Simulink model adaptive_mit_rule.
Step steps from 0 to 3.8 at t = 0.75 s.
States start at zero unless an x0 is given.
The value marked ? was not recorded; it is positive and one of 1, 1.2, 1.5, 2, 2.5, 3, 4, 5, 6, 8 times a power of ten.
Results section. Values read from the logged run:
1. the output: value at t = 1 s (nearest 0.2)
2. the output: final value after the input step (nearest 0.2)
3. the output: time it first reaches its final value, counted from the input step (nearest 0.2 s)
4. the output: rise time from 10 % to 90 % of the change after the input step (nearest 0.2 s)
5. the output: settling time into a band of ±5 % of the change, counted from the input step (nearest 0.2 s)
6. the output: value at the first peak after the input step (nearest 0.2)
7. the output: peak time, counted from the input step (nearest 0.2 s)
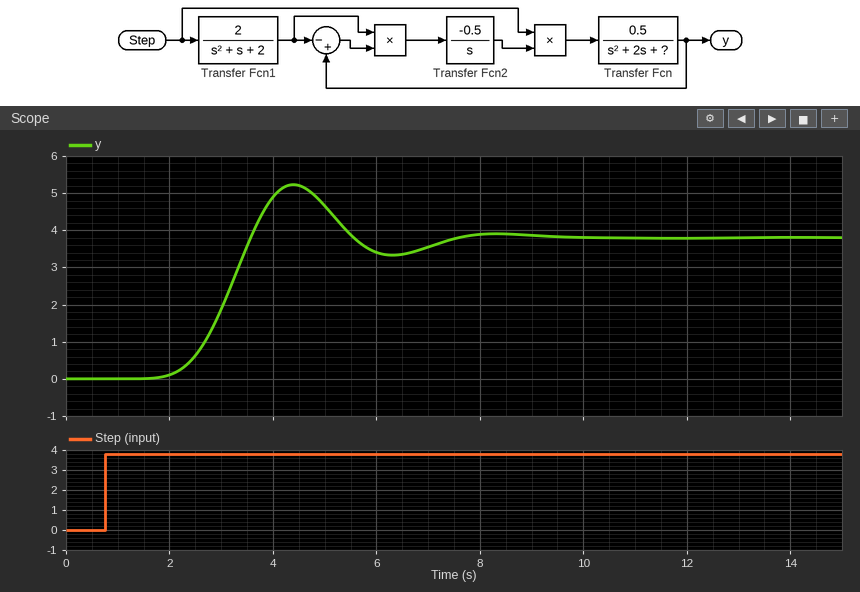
0.0
3.8
2.8 s
1.2 s
6.4 s
5.2
3.6 s
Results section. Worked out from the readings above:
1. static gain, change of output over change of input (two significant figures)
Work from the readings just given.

1.0
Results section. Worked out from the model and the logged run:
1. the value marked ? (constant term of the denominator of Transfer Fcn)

5
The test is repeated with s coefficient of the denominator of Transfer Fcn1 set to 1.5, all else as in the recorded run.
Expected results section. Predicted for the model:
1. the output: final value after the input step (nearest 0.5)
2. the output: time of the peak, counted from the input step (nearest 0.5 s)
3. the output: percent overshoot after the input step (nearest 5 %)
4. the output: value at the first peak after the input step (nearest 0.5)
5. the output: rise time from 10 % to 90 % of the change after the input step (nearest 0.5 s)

4.0
4.0 s
15 %
4.5
1.5 s
